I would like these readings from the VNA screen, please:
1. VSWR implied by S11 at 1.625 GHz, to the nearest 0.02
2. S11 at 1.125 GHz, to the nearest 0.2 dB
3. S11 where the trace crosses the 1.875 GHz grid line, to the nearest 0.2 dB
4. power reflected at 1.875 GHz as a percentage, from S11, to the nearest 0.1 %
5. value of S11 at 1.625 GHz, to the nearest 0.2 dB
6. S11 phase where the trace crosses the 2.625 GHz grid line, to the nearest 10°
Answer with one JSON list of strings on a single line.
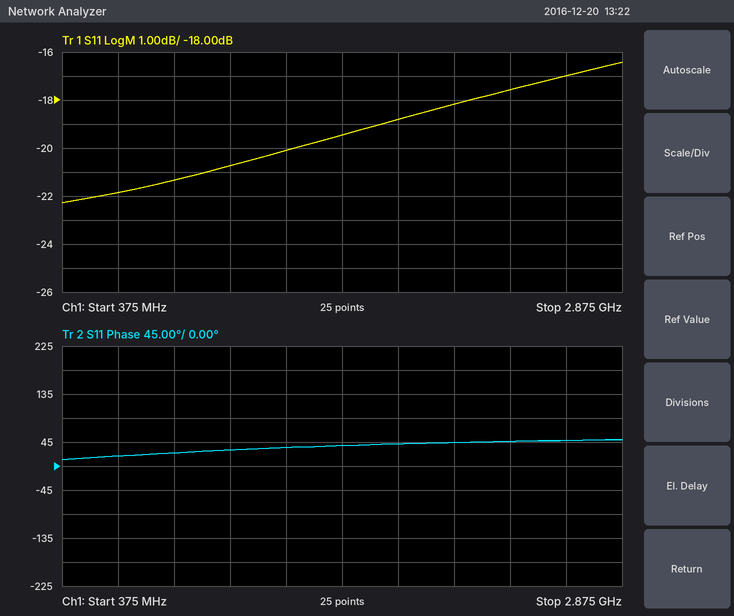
["1.24", "-20.8 dB", "-18.8 dB", "1.3 %", "-19.4 dB", "50°"]
